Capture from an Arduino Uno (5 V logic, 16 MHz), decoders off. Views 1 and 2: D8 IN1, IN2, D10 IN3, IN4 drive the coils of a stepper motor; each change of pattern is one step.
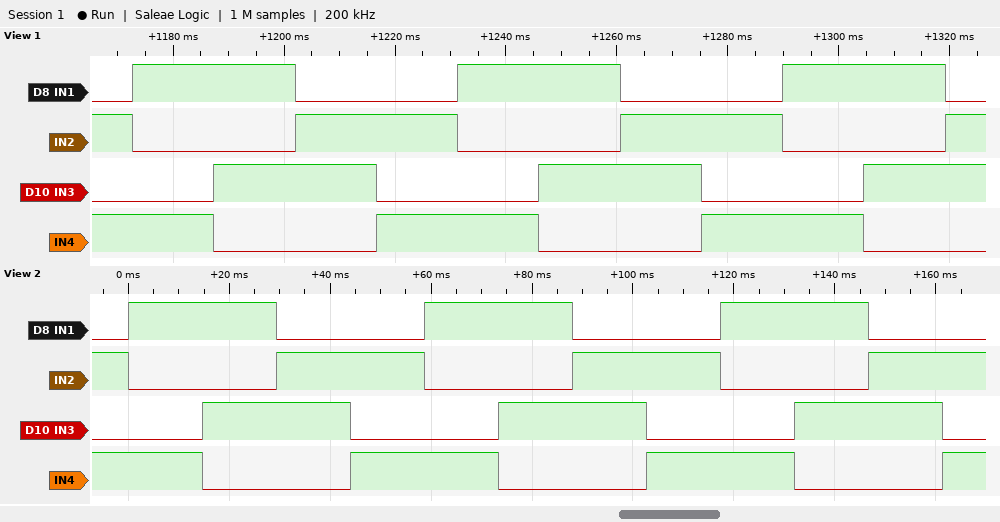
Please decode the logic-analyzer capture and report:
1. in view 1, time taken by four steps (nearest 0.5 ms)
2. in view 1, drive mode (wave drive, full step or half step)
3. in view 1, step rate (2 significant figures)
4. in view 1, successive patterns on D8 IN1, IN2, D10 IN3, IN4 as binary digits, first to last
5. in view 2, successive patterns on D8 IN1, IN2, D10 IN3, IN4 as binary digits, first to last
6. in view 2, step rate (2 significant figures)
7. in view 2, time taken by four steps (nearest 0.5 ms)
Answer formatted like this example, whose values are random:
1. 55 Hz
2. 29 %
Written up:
1. 58.5 ms
2. full step
3. 68 steps/s
4. 0101 1001 1010 0110 0101 1001 1010 0110 0101 1001 1010 0110
5. 0101 1001 1010 0110 0101 1001 1010 0110 0101 1001 1010 0110 0101
6. 68 steps/s
7. 58.5 ms
